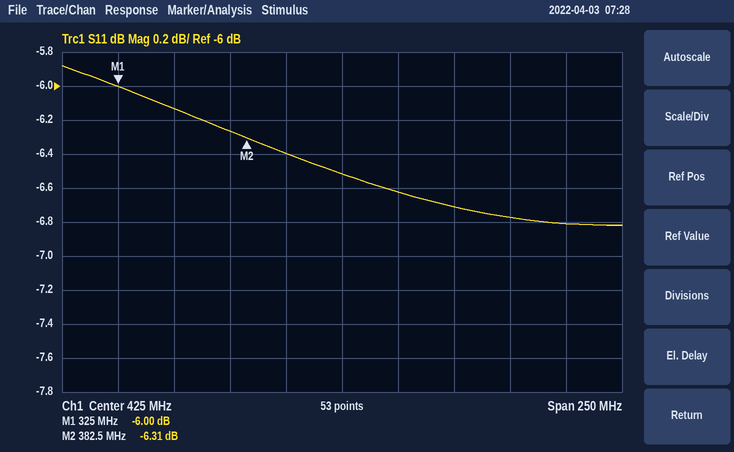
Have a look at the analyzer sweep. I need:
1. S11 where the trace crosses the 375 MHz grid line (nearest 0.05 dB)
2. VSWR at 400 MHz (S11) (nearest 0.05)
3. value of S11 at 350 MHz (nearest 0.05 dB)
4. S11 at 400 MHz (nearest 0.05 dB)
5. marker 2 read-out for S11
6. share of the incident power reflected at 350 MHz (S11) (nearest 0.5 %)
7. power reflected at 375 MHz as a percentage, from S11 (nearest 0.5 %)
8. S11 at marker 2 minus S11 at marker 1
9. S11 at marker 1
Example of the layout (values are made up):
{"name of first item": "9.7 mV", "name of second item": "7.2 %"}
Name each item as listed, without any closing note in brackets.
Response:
{"S11 where the trace crosses the 375 MHz grid line": "-6.25 dB", "VSWR at 400 MHz (S11)": "2.85", "value of S11 at 350 MHz": "-6.15 dB", "S11 at 400 MHz": "-6.40 dB", "marker 2 read-out for S11": "-6.31 dB", "share of the incident power reflected at 350 MHz (S11)": "24.5 %", "power reflected at 375 MHz as a percentage, from S11": "23.5 %", "S11 at marker 2 minus S11 at marker 1": "-0.31 dB", "S11 at marker 1": "-6.00 dB"}
